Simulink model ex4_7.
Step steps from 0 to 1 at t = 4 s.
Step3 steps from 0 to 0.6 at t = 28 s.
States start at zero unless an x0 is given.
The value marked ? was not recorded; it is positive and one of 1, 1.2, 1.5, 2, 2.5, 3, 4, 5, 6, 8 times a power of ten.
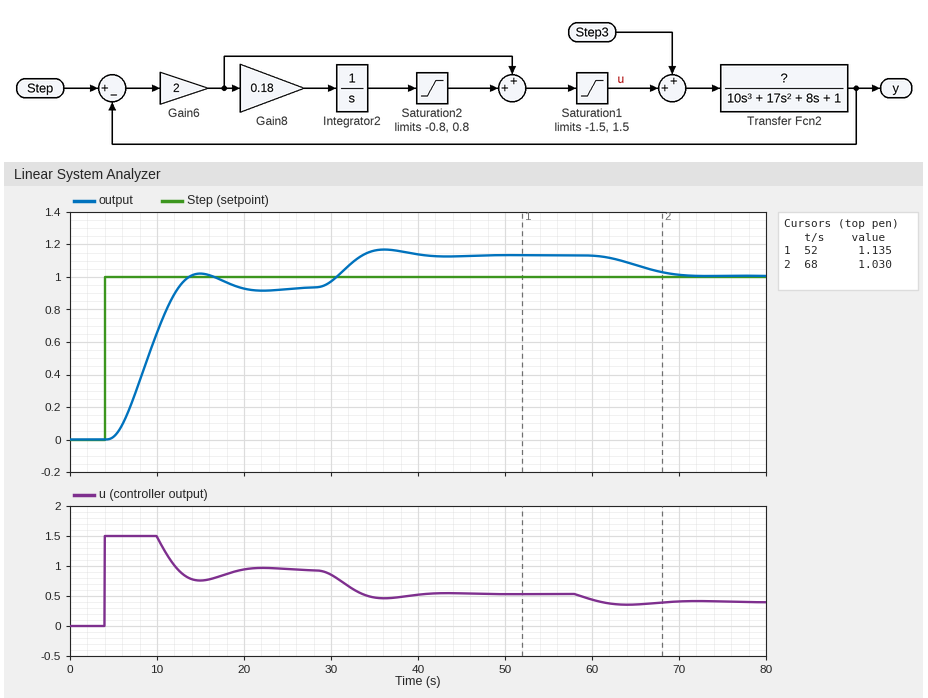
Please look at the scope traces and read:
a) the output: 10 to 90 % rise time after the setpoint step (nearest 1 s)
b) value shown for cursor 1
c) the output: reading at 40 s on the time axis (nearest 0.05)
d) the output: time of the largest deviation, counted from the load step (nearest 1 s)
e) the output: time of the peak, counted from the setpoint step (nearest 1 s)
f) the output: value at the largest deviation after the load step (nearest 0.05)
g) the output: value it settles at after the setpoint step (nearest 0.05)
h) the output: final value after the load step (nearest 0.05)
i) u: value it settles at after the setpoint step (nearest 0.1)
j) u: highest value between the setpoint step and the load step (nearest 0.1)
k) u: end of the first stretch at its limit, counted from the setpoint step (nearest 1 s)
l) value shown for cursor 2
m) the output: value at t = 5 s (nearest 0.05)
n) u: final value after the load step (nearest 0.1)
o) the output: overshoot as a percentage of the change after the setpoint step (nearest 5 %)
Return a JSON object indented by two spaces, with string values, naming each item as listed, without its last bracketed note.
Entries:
{
  "the output: 10 to 90 % rise time after the setpoint step": "5 s",
  "value shown for cursor 1": "1.135",
  "the output: reading at 40 s on the time axis": "1.15",
  "the output: time of the largest deviation, counted from the load step": "8 s",
  "the output: time of the peak, counted from the setpoint step": "11 s",
  "the output: value at the largest deviation after the load step": "1.15",
  "the output: value it settles at after the setpoint step": "0.95",
  "the output: final value after the load step": "1.00",
  "u: value it settles at after the setpoint step": "0.9",
  "u: highest value between the setpoint step and the load step": "1.5",
  "u: end of the first stretch at its limit, counted from the setpoint step": "6 s",
  "value shown for cursor 2": "1.030",
  "the output: value at t = 5 s": "0.00",
  "u: final value after the load step": "0.4",
  "the output: overshoot as a percentage of the change after the setpoint step": "10 %"
}
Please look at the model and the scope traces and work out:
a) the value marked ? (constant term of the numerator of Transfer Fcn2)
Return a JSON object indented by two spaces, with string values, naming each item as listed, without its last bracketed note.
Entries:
{
  "the value marked ?": "1"
}
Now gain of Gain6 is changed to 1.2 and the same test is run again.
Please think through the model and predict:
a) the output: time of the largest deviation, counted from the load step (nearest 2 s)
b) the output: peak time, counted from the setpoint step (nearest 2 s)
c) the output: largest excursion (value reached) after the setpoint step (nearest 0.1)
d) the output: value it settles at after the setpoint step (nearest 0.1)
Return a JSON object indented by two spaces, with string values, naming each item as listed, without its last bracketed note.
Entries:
{
  "the output: time of the largest deviation, counted from the load step": "10 s",
  "the output: peak time, counted from the setpoint step": "12 s",
  "the output: largest excursion (value reached) after the setpoint step": "1.0",
  "the output: value it settles at after the setpoint step": "0.9"
}
